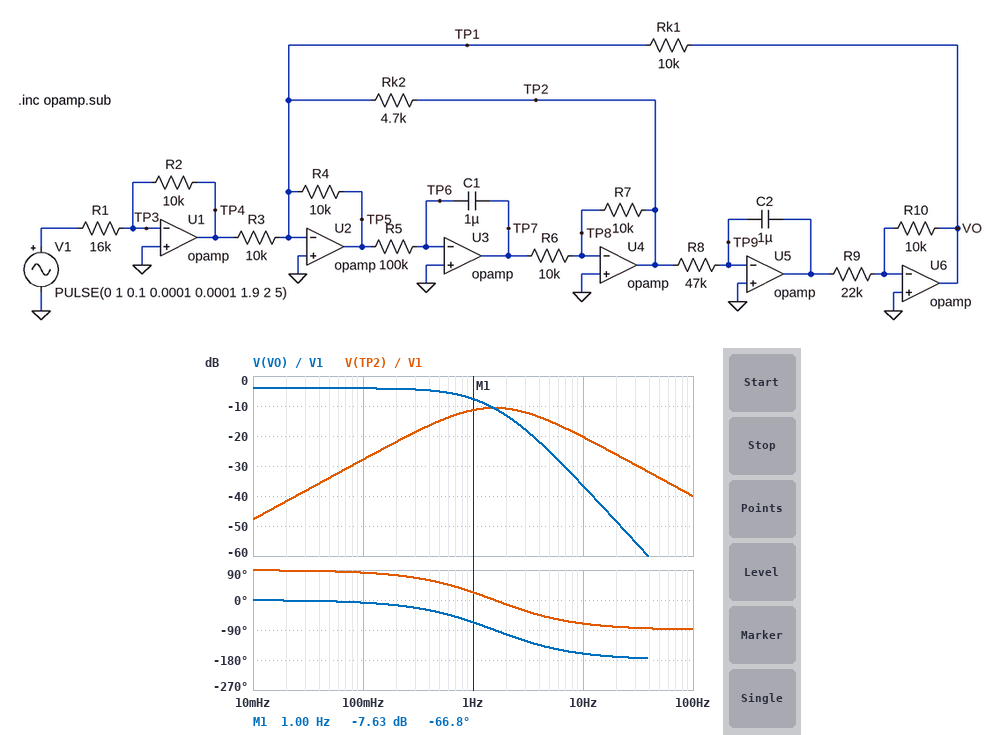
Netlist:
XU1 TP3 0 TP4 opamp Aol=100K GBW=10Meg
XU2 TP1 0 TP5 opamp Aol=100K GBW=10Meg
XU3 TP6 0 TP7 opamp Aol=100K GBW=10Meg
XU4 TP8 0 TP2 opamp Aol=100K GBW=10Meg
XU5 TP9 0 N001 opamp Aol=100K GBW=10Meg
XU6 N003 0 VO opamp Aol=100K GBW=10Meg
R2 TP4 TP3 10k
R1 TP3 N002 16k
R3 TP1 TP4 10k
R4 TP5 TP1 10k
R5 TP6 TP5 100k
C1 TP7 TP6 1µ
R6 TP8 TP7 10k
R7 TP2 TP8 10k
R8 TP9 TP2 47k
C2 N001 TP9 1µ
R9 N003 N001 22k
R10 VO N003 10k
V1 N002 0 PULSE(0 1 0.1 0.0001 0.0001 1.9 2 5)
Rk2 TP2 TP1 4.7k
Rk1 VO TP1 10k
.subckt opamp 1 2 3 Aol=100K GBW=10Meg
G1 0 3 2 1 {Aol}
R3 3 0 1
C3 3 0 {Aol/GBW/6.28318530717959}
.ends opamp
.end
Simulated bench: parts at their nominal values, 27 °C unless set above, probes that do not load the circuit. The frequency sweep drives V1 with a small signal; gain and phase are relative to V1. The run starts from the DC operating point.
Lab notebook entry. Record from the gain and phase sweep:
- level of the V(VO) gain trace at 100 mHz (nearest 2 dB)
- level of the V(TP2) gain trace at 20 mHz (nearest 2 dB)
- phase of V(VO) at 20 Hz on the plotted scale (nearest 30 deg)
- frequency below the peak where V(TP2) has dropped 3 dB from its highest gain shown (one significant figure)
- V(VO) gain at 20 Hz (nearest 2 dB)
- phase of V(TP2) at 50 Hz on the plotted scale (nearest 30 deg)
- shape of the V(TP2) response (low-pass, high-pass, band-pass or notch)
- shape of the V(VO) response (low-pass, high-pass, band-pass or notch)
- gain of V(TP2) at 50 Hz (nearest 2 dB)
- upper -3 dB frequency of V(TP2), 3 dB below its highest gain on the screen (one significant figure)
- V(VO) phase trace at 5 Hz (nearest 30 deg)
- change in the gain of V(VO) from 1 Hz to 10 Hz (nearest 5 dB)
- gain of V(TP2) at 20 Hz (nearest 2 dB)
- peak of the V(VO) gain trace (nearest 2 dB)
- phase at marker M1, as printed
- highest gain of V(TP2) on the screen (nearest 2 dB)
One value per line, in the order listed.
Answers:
-4 dB
-42 dB
-180 deg
600 mHz
-48 dB
-90 deg
band-pass
low-pass
-34 dB
4 Hz
-150 deg
-30 dB
-26 dB
-4 dB
-66.8 deg
-10 dB
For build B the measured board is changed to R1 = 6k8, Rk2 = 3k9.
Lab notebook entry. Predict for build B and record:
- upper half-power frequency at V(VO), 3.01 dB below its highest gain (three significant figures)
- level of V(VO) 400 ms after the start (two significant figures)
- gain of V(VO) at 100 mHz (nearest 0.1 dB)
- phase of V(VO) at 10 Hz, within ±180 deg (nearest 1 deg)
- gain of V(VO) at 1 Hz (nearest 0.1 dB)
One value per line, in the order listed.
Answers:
700 mHz
1.0 V
3.3 dB
-157 deg
-1.6 dB
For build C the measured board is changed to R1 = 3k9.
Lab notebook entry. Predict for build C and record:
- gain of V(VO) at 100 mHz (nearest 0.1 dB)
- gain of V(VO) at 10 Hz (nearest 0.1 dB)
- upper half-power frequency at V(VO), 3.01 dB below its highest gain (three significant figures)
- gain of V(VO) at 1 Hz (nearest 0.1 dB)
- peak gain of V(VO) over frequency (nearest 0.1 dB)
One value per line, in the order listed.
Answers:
8.1 dB
-24.3 dB
902 mHz
4.6 dB
8.2 dB
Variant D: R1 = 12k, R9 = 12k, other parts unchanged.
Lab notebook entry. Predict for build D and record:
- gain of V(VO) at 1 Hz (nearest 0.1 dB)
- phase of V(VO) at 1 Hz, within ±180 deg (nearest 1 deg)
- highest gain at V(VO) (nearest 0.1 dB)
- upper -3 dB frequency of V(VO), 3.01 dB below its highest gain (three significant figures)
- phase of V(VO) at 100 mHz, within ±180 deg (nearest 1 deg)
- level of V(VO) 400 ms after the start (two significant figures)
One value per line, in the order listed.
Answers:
-2.3 dB
-44 deg
-1.6 dB
1.85 Hz
-4 deg
830 mV
